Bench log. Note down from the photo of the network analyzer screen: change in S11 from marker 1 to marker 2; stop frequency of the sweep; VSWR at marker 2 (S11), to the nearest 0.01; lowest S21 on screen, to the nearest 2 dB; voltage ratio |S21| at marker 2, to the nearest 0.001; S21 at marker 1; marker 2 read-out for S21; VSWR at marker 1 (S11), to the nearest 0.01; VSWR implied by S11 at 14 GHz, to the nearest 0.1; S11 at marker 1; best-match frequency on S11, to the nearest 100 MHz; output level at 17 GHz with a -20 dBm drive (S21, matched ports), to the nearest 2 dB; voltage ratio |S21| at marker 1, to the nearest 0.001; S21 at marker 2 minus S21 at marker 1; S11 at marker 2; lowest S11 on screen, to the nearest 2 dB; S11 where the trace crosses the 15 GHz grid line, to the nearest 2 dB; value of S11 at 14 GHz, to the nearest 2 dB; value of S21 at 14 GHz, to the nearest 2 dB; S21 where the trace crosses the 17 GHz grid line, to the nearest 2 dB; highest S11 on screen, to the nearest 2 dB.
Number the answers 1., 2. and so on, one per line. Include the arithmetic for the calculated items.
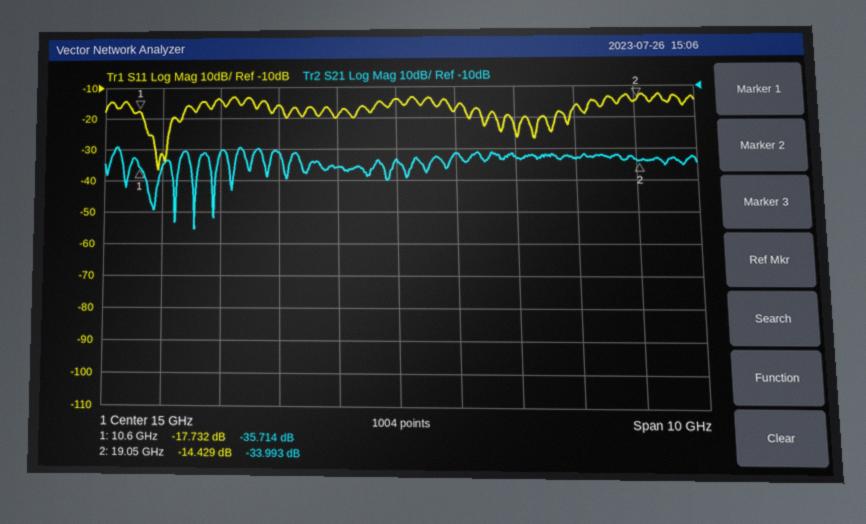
1. -14.429 − (-17.732) = 3.303 dB
2. 20 GHz
3. (1 + 0.1899)/(1 − 0.1899) ≈ 1.47
4. -56 dB
5. 10^(-33.993/20) ≈ 0.020
6. -35.714 dB
7. -33.993 dB
8. (1 + 0.1298)/(1 − 0.1298) ≈ 1.30
9. |Γ| = 10^(-20/20) = 0.1000; VSWR = (1 + 0.1000)/(1 − 0.1000) ≈ 1.2
10. -17.732 dB
11. 10.9 GHz
12. -20 dBm + (-32 dB) = -52 dBm
13. 10^(-35.714/20) ≈ 0.016
14. -33.993 − (-35.714) = 1.721 dB
15. -14.429 dB
16. -36 dB
17. -14 dB
18. -20 dB
19. -36 dB
20. -32 dB
21. -12 dB
